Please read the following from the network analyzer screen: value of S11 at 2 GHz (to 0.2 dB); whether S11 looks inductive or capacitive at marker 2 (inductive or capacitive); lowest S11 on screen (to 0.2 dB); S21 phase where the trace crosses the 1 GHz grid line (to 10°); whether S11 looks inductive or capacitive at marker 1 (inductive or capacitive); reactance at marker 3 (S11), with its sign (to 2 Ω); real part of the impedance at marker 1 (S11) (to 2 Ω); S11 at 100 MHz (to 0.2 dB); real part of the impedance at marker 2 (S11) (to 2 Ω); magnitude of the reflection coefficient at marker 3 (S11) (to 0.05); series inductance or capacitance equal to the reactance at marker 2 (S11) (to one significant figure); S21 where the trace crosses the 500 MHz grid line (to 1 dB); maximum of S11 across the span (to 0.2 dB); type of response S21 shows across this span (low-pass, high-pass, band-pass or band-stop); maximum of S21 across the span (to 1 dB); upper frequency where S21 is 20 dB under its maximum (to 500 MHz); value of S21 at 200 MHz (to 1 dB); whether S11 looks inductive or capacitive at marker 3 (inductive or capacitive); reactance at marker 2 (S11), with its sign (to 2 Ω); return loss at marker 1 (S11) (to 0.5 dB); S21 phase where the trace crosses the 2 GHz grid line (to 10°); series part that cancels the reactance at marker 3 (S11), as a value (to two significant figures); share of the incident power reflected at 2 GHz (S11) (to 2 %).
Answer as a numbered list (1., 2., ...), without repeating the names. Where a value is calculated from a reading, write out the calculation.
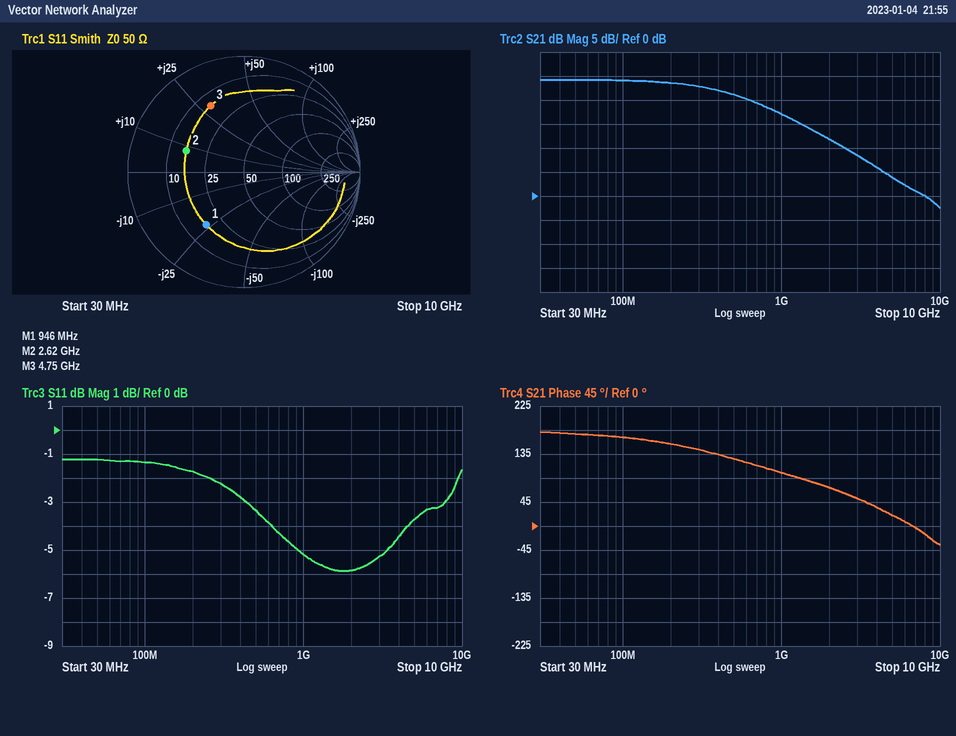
1. -5.8 dB
2. inductive
3. -5.8 dB
4. 100°
5. capacitive
6. +28 Ω
7. 18 Ω
8. -1.4 dB
9. 16 Ω
10. 0.65
11. L = 8 Ω/(2π × 2.62 GHz) ≈ 486 pH, so 500 pH to one significant figure
12. 21 dB
13. -1.2 dB
14. low-pass
15. 24 dB
16. 5.0 GHz
17. 24 dB
18. inductive
19. +8 Ω
20. 5.0 dB
21. 70°
22. C = 1/(2π × 4.75 GHz × 28 Ω) ≈ 1.2 pF
23. 10^(-5.8/10) ≈ 26 %
